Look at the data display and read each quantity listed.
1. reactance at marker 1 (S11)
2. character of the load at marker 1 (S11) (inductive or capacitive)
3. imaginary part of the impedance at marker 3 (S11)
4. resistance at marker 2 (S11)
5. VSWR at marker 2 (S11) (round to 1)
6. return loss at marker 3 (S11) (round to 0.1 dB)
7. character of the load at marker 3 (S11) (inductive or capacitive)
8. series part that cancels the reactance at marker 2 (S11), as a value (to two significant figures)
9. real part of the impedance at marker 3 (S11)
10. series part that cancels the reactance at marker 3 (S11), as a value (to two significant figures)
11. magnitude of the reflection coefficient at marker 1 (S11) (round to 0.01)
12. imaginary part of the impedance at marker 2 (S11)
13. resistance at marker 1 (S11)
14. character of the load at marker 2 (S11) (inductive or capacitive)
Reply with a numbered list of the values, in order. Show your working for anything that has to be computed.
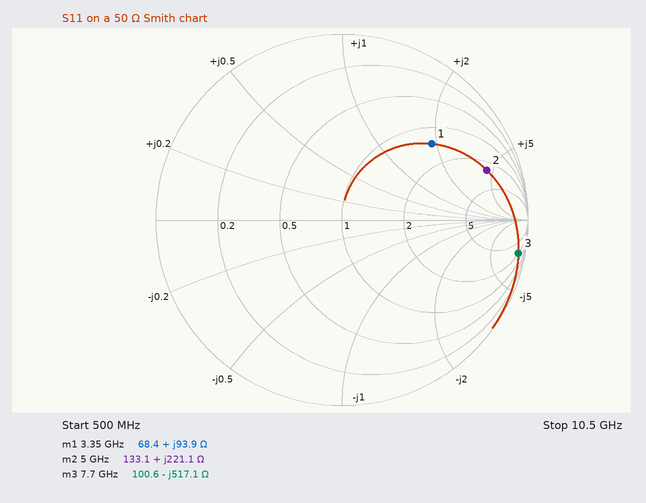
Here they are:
1. +93.9 Ω
2. inductive
3. -517.1 Ω
4. 133.1 Ω
5. 10
6. 0.3 dB
7. capacitive
8. C = 1/(2π × 5 GHz × 221.1 Ω) ≈ 144 fF, so 140 fF to two significant figures
9. 100.6 Ω
10. L = 517.1 Ω/(2π × 7.7 GHz) ≈ 11 nH
11. 0.63
12. +221.1 Ω
13. 68.4 Ω
14. inductive
